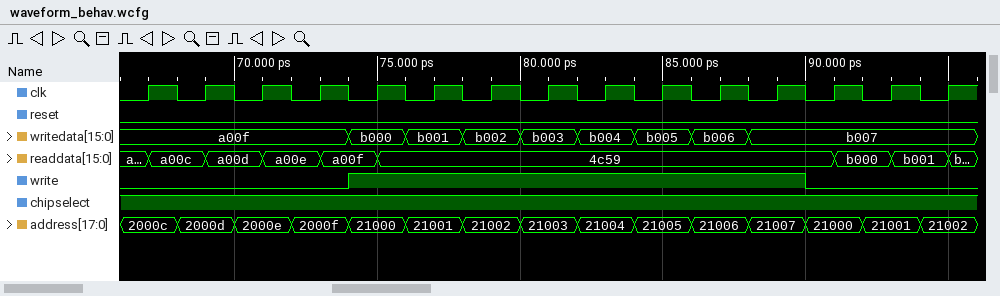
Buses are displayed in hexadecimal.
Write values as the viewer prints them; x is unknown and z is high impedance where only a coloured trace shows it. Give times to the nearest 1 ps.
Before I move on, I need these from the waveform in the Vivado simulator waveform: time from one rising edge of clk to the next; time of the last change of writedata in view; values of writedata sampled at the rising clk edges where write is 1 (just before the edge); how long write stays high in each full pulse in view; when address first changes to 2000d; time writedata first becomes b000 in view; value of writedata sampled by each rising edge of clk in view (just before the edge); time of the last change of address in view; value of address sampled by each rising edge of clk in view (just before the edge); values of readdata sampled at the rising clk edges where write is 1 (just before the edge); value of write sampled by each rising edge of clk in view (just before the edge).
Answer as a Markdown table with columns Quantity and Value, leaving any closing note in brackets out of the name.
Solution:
| Quantity | Value |
|---|---|
| time from one rising edge of clk to the next | 2 ps |
| time of the last change of writedata in view | 88 ps |
| values of writedata sampled at the rising clk edges where write is 1 | b000, b001, b002, b003, b004, b005, b006, b007 |
| how long write stays high in each full pulse in view | 16 ps |
| when address first changes to 2000d | 68 ps |
| time writedata first becomes b000 in view | 74 ps |
| value of writedata sampled by each rising edge of clk in view | a00f, a00f, a00f, a00f, b000, b001, b002, b003, b004, b005, b006, b007, b007, b007, b007 |
| time of the last change of address in view | 94 ps |
| value of address sampled by each rising edge of clk in view | 2000c, 2000d, 2000e, 2000f, 21000, 21001, 21002, 21003, 21004, 21005, 21006, 21007, 21000, 21001, 21002 |
| values of readdata sampled at the rising clk edges where write is 1 | a00f, 4c59, 4c59, 4c59, 4c59, 4c59, 4c59, 4c59 |
| value of write sampled by each rising edge of clk in view | 0 0 0 0 1 1 1 1 1 1 1 1 0 0 0 |
